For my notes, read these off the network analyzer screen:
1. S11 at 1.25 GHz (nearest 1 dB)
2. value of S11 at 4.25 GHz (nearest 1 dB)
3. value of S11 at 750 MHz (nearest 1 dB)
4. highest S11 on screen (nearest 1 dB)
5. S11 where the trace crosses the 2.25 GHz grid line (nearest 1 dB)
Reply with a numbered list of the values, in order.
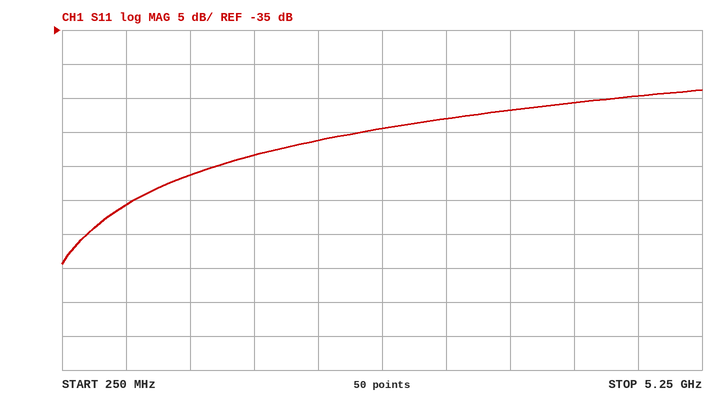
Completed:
1. -56 dB
2. -46 dB
3. -61 dB
4. -44 dB
5. -51 dB
